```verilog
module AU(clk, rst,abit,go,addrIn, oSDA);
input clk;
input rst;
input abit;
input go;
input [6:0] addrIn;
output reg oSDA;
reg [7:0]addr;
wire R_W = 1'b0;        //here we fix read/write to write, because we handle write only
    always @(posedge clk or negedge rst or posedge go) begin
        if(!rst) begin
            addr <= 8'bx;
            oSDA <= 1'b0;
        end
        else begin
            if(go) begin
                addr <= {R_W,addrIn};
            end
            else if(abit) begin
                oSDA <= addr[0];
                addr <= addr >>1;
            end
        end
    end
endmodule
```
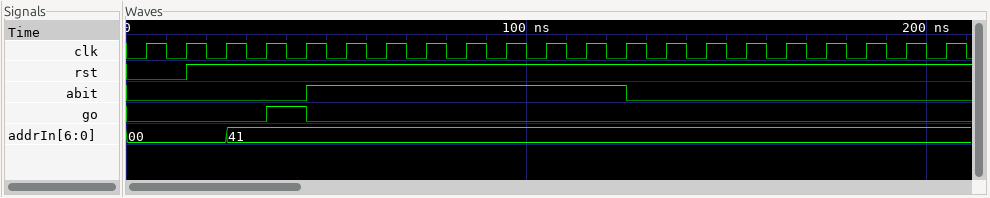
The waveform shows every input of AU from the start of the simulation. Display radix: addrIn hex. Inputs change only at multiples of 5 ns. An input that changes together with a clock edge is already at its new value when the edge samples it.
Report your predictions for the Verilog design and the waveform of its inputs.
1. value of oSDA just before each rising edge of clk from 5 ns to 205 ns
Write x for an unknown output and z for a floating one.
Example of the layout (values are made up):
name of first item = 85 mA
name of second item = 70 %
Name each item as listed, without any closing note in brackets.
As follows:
value of oSDA just before each rising edge of clk from 5 ns to 205 ns = 0 0 0 0 0 1 0 0 0 0 0 1 0 0 0 0 0 0 0 0 0
